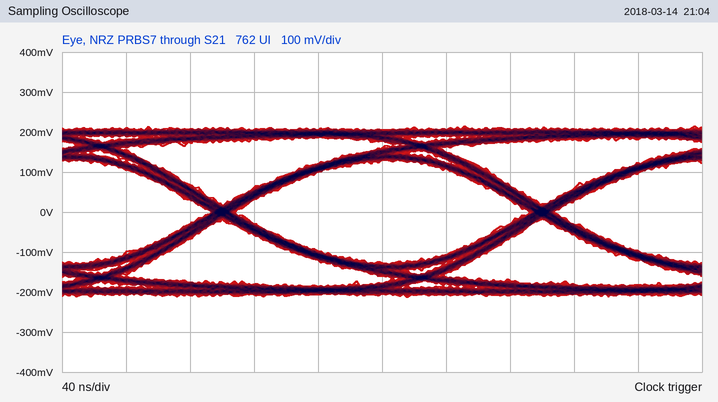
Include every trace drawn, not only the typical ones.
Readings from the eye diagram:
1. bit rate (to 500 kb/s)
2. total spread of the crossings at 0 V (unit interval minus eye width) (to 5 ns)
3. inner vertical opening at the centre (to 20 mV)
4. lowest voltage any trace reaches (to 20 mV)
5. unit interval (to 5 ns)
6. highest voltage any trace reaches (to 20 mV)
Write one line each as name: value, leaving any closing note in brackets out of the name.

bit rate: 5.0 Mb/s
total spread of the crossings at 0 V (unit interval minus eye width): 15 ns
inner vertical opening at the centre: 260 mV
lowest voltage any trace reaches: -220 mV
unit interval: 200 ns
highest voltage any trace reaches: 220 mV
